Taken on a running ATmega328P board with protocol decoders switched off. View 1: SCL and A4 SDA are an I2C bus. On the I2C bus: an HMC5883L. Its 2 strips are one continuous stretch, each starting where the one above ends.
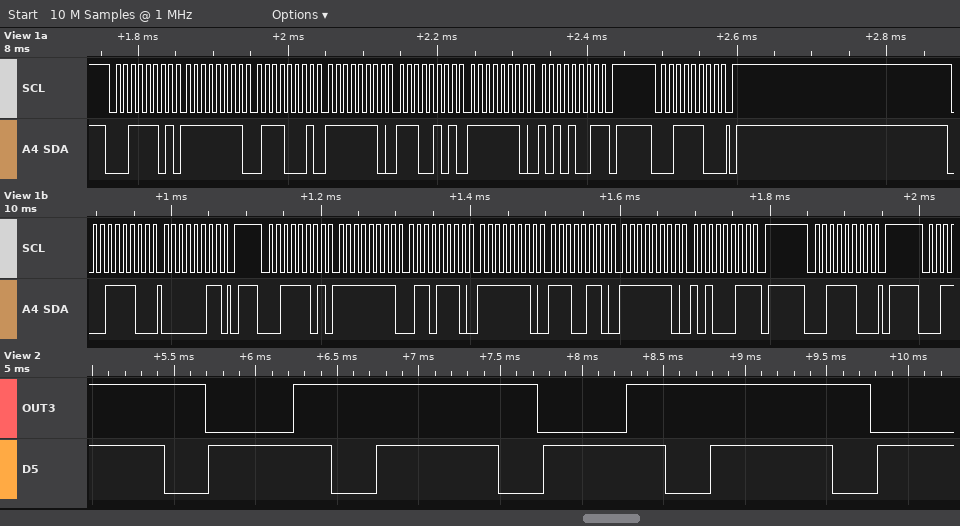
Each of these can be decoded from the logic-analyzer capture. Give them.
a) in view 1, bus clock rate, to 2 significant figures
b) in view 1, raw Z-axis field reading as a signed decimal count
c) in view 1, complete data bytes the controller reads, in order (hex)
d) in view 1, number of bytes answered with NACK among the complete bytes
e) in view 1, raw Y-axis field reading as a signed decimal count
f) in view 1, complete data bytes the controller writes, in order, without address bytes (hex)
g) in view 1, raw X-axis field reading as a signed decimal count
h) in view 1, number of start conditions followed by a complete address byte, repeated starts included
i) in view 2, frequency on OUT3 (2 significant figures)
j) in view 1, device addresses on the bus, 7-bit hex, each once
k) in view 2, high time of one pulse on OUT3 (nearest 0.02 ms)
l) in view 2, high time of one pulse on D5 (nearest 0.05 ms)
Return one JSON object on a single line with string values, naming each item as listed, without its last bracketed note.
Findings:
{"in view 1, bus clock rate, to 2 significant figures": "100 kHz", "in view 1, raw Z-axis field reading as a signed decimal count": "-282", "in view 1, complete data bytes the controller reads, in order": "FF 71 FE E5 FE A9 FF 6E FE E6 FE A3", "in view 1, number of bytes answered with NACK among the complete bytes": "2", "in view 1, raw Y-axis field reading as a signed decimal count": "-349", "in view 1, complete data bytes the controller writes, in order, without address bytes": "03", "in view 1, raw X-axis field reading as a signed decimal count": "-146", "in view 1, number of start conditions followed by a complete address byte, repeated starts included": "5", "in view 2, frequency on OUT3": "490 Hz", "in view 1, device addresses on the bus, 7-bit hex, each once": "0x1E", "in view 2, high time of one pulse on OUT3": "1.50 ms", "in view 2, high time of one pulse on D5": "0.75 ms"}
